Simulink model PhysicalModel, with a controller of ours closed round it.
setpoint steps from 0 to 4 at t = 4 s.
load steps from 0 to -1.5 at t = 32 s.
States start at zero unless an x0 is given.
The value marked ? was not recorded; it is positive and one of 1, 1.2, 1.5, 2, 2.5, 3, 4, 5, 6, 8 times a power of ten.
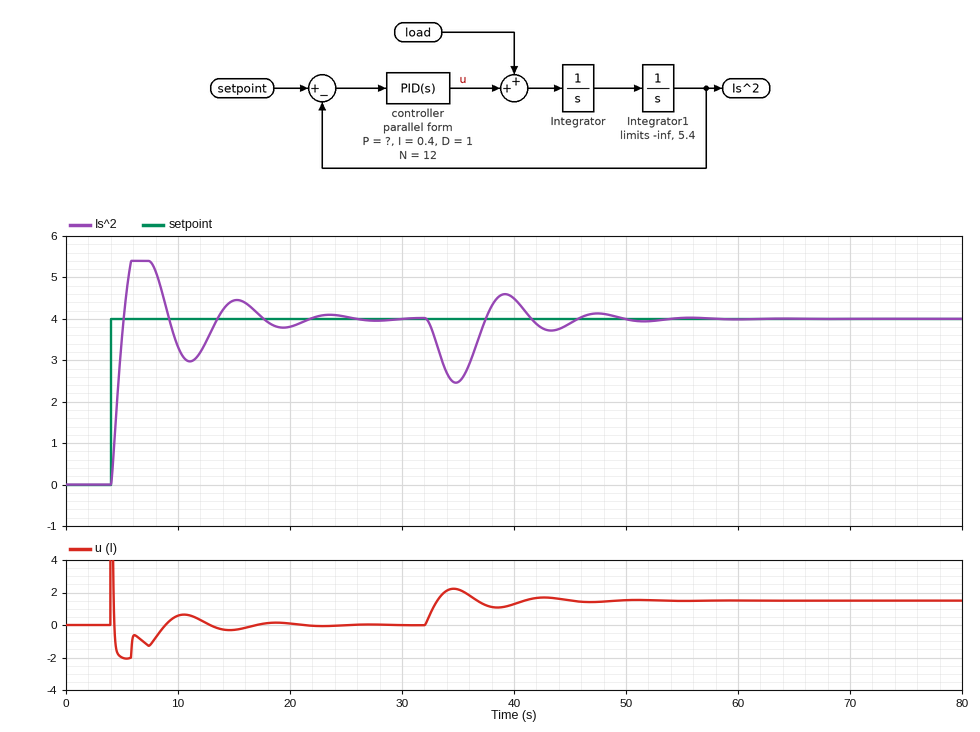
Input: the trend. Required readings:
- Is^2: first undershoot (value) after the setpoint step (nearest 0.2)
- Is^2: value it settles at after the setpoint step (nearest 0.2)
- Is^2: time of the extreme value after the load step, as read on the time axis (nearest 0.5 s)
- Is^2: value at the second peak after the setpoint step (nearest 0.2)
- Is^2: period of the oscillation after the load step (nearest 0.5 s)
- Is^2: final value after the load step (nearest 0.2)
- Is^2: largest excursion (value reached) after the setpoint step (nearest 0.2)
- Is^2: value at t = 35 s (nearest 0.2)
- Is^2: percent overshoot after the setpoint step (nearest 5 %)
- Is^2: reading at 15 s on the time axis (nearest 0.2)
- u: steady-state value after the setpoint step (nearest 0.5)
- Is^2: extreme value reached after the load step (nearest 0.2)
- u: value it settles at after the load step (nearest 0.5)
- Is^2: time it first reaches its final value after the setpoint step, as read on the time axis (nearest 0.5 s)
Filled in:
3.0
4.0
35.0 s
4.4
8.5 s
4.0
5.4
2.4
35 %
4.4
0.0
2.4
1.5
5.0 s
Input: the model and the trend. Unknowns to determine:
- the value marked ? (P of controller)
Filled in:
0.8
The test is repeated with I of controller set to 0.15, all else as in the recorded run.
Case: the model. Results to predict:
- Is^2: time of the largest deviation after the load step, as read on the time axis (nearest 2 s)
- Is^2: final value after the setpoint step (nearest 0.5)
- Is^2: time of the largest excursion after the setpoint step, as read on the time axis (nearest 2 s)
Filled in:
36 s
4.0
6 s
